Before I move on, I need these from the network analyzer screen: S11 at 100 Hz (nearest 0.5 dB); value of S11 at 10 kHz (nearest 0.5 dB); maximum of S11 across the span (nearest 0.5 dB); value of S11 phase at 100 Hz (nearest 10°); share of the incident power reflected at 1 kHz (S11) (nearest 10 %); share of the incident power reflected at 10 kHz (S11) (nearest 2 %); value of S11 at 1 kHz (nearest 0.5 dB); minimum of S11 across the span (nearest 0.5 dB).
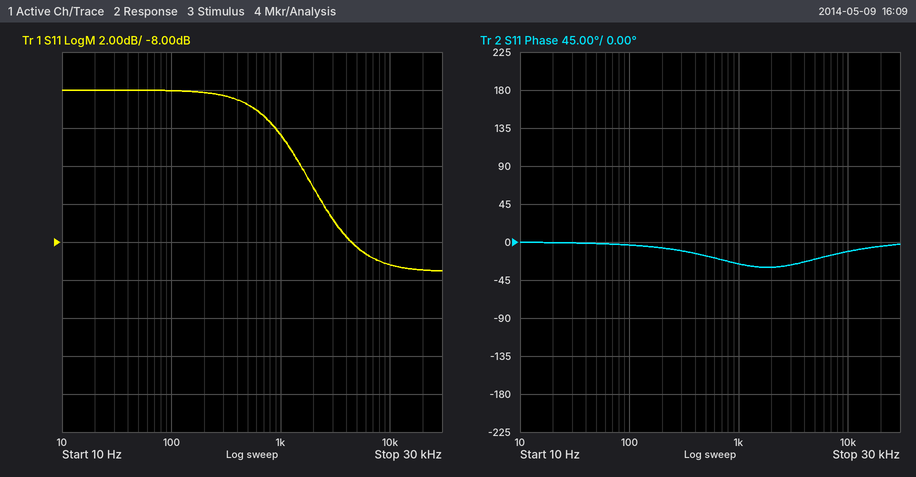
0.0 dB
-9.0 dB
0.0 dB
0°
60 %
12 %
-2.5 dB
-9.5 dB
